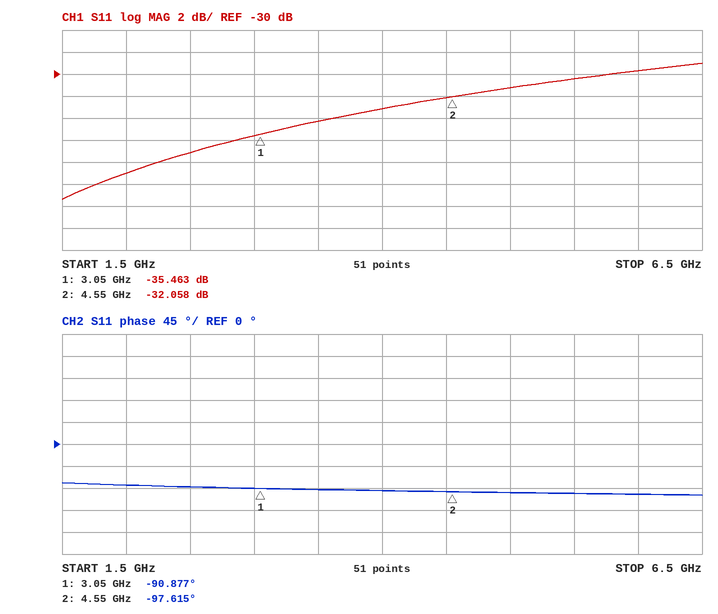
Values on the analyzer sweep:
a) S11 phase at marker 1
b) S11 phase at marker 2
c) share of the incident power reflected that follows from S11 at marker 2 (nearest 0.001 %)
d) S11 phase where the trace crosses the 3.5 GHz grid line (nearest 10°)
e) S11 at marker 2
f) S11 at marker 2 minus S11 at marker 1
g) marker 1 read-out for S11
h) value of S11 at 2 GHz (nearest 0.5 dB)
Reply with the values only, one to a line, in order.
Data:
-90.877°
-97.615°
0.062 %
-90°
-32.058 dB
3.405 dB
-35.463 dB
-39.0 dB
